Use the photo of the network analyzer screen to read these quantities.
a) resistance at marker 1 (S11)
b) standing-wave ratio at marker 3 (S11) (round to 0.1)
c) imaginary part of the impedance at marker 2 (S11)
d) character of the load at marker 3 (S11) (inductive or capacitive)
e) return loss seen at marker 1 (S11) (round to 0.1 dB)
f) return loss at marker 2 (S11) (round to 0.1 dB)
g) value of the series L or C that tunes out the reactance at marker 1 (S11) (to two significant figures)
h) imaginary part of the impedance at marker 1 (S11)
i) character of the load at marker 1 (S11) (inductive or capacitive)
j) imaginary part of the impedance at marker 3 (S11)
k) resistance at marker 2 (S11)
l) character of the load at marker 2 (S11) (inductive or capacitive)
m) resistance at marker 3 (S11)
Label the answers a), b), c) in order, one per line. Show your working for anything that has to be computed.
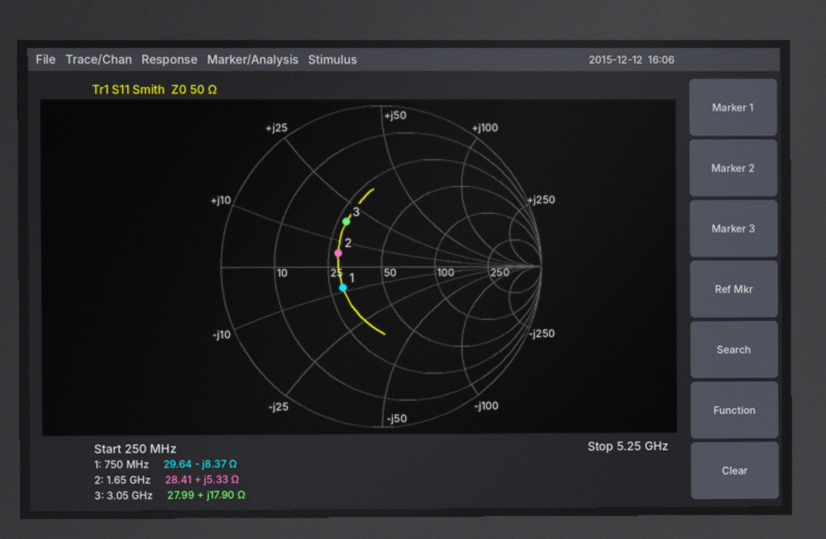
a) 29.64 Ω
b) 2.1
c) +5.33 Ω
d) inductive
e) 11.2 dB
f) 11.0 dB
g) L = 8.37 Ω/(2π × 750 MHz) ≈ 1.8 nH
h) -8.37 Ω
i) capacitive
j) +17.90 Ω
k) 28.41 Ω
l) inductive
m) 27.99 Ω
